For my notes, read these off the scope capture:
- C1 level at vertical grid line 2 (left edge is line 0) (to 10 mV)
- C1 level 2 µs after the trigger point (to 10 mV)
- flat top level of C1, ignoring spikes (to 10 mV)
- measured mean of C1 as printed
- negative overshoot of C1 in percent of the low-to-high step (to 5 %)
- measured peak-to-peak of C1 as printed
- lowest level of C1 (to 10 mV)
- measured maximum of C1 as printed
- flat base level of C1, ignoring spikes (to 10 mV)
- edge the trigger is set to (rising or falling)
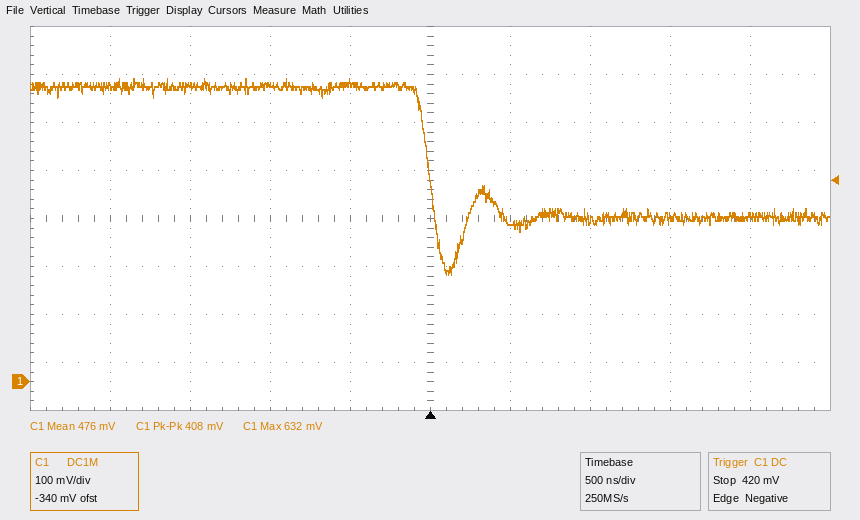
620 mV
340 mV
620 mV
476 mV
45 %
408 mV
220 mV
632 mV
340 mV
falling
